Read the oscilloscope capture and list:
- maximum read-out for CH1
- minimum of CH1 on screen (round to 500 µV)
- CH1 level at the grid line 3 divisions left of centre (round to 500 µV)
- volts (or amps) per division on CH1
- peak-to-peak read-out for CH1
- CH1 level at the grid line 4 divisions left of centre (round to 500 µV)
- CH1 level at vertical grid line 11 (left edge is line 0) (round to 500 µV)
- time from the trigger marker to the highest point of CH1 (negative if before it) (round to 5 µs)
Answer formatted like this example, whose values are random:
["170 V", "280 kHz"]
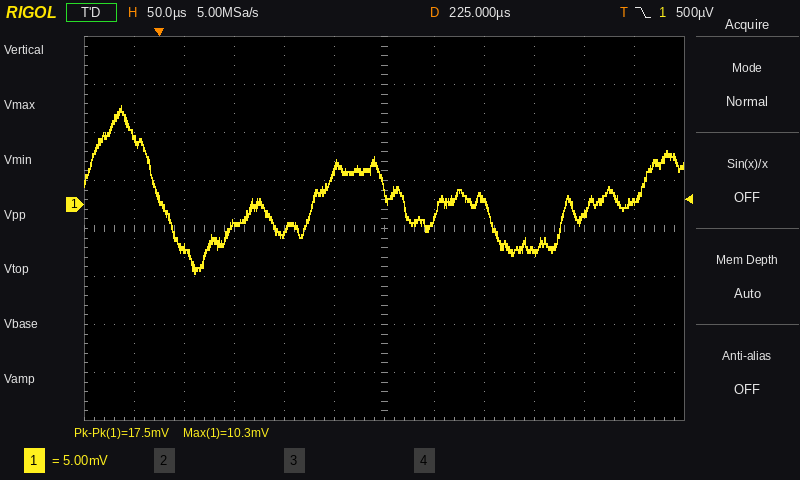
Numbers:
["10.3 mV", "-7.0 mV", "-2.0 mV", "5 mV", "17.5 mV", "-4.5 mV", "500 µV", "-40 µs"]
